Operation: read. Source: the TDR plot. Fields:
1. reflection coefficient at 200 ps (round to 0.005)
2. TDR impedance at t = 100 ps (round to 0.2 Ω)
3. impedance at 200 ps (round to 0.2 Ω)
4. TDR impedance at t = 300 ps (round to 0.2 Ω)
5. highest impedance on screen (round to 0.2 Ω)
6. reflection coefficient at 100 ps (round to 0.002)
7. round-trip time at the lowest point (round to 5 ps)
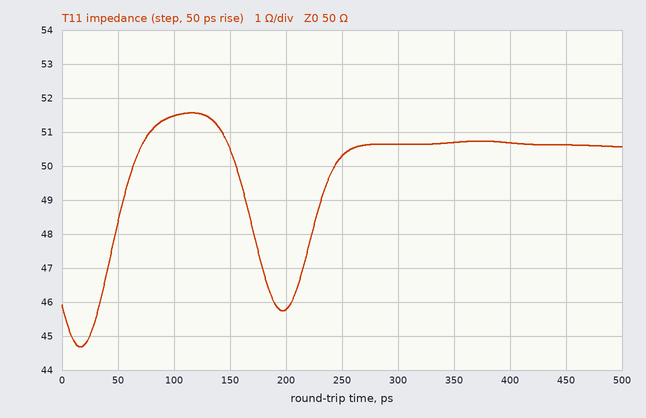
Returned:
-0.045
51.4 Ω
45.8 Ω
50.6 Ω
51.6 Ω
+0.014
15 ps
